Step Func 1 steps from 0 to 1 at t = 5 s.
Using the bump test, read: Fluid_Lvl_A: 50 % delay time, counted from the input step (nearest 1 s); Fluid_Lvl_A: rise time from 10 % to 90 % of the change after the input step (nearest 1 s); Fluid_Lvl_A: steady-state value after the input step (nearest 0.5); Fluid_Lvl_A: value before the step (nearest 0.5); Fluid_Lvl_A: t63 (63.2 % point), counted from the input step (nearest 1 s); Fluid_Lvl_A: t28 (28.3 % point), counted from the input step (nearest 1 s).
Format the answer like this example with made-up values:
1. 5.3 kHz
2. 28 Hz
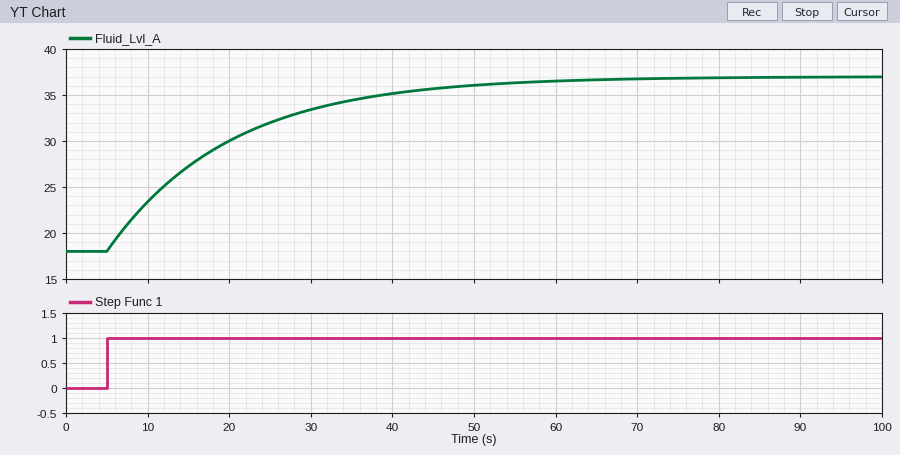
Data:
1. 10 s
2. 33 s
3. 37.0
4. 18.0
5. 15 s
6. 5 s
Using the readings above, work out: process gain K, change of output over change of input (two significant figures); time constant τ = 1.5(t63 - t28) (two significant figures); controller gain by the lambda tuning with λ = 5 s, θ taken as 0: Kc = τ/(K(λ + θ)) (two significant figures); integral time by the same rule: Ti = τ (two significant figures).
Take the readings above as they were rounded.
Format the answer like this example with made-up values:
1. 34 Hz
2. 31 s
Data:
1. 19
2. 15 s
3. 0.16
4. 15 s
